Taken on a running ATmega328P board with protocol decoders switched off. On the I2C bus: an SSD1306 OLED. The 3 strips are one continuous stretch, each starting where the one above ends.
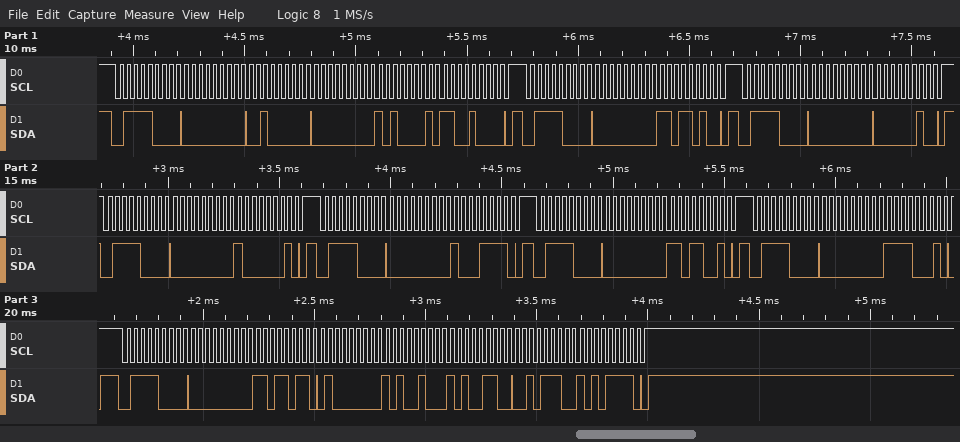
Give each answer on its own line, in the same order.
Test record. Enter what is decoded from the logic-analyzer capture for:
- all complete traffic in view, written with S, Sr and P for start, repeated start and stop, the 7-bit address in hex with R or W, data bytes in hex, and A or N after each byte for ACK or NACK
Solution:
S 3CW A 00 A 20 A 00 A A1 A C8 A P S 3CW A 00 A DA A P S 3CW A 00 A 02 A P S 3CW A 00 A 81 A P S 3CW A 00 A 8F A P S 3CW A 00 A D9 A P S 3CW A 00 A F1 A P S 3CW A 00 A DB A 40 A A4 A A6 A 2E A AF A P
